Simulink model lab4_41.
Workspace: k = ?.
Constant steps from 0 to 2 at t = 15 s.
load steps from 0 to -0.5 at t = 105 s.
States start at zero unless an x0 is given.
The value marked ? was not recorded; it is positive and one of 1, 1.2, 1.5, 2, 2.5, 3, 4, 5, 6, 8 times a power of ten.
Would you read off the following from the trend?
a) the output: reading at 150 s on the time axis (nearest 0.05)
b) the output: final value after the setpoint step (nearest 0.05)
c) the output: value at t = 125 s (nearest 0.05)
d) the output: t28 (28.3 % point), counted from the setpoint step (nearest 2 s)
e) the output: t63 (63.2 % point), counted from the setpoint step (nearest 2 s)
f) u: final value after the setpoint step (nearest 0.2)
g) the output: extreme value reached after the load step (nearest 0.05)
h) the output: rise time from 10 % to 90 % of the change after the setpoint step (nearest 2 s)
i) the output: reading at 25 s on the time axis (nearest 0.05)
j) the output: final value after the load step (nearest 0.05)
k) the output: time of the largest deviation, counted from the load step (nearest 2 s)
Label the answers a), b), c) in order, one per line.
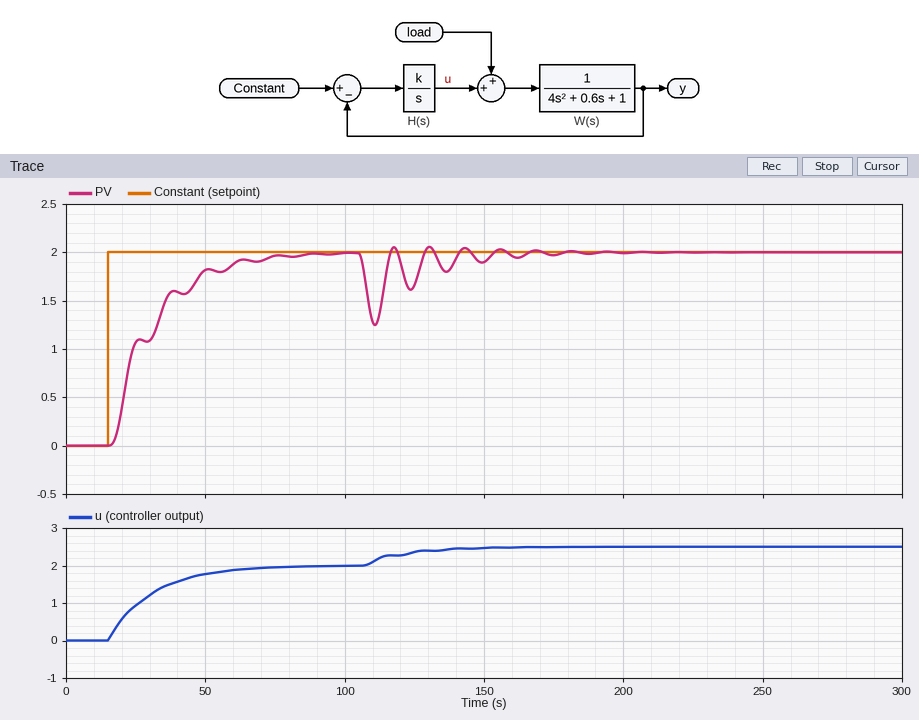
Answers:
a) 1.90
b) 2.00
c) 1.65
d) 6 s
e) 18 s
f) 2.0
g) 1.25
h) 30 s
i) 1.05
j) 2.00
k) 6 s
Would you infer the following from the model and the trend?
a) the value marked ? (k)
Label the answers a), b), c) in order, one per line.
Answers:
a) 0.06
